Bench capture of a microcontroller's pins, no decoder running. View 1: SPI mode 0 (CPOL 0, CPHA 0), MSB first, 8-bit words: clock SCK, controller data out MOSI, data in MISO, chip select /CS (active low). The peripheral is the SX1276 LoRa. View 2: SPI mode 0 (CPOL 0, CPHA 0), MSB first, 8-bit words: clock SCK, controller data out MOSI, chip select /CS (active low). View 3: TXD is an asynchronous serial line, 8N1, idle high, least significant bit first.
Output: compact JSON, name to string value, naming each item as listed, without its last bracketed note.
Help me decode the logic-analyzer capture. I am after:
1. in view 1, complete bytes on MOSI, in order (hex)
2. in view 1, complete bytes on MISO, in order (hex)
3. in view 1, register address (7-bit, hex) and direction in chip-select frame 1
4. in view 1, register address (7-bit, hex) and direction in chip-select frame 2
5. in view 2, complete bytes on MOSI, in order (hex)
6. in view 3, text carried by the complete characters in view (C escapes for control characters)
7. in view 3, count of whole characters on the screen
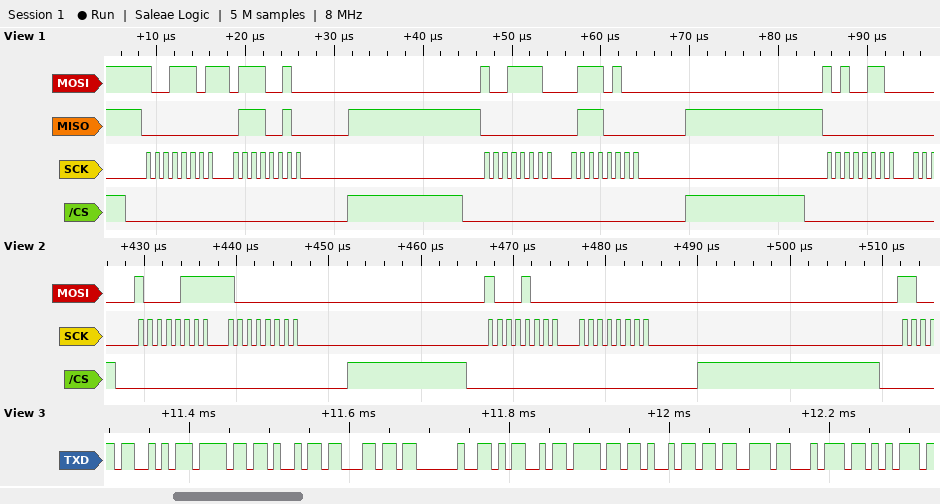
{"in view 1, complete bytes on MOSI, in order": "0x9D 0x72 0x9E 0x74 0xA6", "in view 1, complete bytes on MISO, in order": "0x00 0x72 0x00 0x70 0x00", "in view 1, register address (7-bit, hex) and direction in chip-select frame 1": "0x1D write", "in view 1, register address (7-bit, hex) and direction in chip-select frame 2": "0x1E write", "in view 2, complete bytes on MOSI, in order": "87 80 88 00", "in view 3, text carried by the complete characters in view": "\"Soil Moistu\"", "in view 3, count of whole characters on the screen": "11"}
